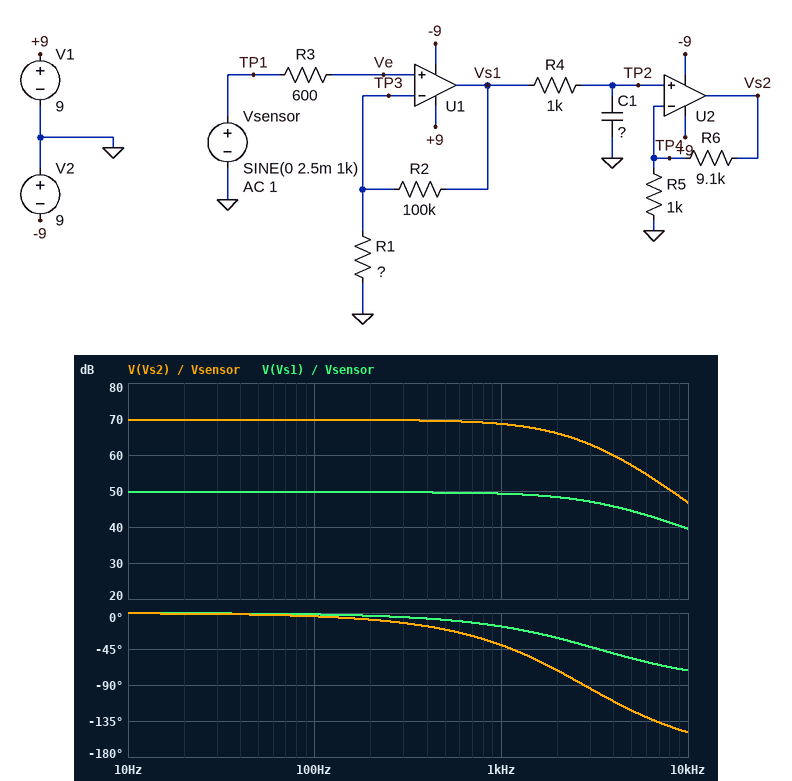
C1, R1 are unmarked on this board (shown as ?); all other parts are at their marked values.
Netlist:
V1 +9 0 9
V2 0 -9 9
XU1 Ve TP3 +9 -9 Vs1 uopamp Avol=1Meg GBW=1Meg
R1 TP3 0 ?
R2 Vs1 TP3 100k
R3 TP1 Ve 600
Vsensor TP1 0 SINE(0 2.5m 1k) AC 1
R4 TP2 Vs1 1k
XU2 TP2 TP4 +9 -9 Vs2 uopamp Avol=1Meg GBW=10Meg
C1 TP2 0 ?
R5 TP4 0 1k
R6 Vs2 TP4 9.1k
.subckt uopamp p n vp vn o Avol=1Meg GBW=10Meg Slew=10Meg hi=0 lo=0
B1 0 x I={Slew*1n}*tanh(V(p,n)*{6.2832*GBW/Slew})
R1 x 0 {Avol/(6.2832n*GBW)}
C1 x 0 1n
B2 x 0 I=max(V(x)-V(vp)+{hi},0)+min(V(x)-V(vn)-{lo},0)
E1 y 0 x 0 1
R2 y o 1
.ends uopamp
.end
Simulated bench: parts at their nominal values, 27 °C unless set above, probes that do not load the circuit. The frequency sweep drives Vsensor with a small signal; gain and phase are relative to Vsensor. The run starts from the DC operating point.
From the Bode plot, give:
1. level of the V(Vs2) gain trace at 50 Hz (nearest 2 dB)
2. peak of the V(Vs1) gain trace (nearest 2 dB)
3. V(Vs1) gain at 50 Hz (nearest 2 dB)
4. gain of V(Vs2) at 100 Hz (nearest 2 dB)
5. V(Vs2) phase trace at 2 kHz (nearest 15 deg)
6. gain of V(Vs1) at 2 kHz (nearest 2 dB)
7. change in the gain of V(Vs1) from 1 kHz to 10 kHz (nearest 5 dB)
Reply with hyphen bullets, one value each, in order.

- 70 dB
- 50 dB
- 50 dB
- 70 dB
- -75 deg
- 48 dB
- -10 dB
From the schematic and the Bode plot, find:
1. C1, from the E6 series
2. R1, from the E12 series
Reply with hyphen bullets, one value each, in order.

- 68 nF
- 330 Ω
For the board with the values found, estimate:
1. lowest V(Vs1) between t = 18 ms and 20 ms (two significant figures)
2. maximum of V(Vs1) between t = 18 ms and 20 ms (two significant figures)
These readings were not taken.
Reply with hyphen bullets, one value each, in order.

- -730 mV
- 730 mV
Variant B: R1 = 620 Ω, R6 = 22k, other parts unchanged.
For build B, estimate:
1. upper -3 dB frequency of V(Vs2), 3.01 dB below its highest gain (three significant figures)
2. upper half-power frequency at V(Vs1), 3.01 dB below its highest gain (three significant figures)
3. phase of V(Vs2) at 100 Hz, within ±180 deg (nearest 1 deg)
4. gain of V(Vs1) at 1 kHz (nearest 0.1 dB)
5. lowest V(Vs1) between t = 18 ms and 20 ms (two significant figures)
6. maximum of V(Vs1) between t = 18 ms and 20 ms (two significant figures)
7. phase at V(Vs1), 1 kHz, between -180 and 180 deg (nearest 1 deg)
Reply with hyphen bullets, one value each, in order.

- 2.09 kHz
- 6.16 kHz
- -3 deg
- 44.1 dB
- -400 mV
- 400 mV
- -9 deg
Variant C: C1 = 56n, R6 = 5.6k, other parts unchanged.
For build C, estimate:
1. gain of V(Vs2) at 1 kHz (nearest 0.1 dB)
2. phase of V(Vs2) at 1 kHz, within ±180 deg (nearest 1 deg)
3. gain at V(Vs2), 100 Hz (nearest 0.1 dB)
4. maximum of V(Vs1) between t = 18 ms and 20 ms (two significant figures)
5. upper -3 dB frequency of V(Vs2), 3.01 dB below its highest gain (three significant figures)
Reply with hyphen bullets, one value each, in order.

- 65.2 dB
- -36 deg
- 66.0 dB
- 730 mV
- 1.96 kHz
